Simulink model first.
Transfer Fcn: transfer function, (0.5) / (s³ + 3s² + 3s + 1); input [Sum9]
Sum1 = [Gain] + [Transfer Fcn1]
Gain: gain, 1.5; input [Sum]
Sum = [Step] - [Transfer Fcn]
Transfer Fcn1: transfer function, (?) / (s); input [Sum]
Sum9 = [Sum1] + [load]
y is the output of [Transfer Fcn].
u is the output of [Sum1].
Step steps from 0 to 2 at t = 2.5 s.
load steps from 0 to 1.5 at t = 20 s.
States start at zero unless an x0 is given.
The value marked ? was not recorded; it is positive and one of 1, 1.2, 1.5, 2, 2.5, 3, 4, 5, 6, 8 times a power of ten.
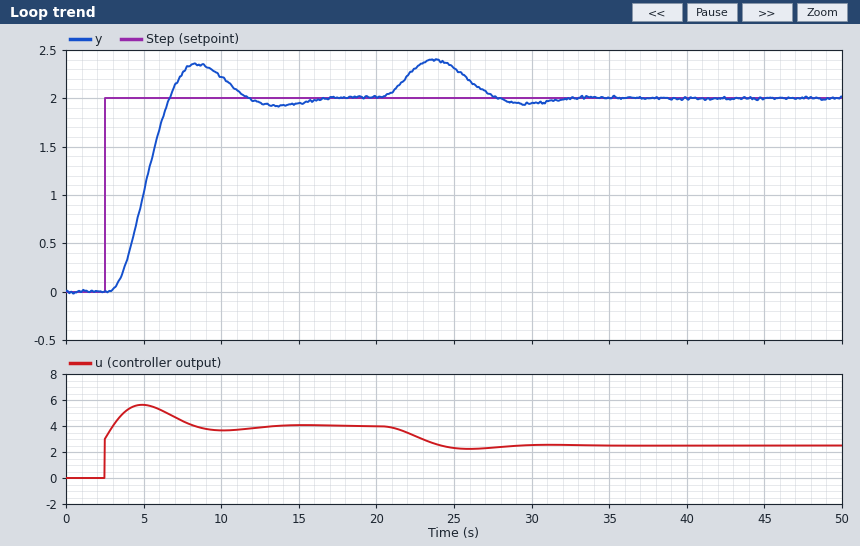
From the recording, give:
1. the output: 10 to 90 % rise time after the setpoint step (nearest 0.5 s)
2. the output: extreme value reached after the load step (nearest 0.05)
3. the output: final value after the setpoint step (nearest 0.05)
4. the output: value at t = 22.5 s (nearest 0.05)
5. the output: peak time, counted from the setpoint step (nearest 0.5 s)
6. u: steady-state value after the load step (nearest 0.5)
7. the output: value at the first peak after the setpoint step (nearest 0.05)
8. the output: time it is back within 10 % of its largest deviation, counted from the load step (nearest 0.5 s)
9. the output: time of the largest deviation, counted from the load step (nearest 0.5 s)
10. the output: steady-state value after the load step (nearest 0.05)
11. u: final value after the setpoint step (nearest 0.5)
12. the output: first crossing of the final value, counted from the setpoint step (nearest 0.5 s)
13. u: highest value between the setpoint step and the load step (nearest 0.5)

2.5 s
2.40
2.00
2.30
6.0 s
2.5
2.35
11.0 s
3.5 s
2.00
4.0
4.0 s
5.5
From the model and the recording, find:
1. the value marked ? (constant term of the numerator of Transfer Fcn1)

1
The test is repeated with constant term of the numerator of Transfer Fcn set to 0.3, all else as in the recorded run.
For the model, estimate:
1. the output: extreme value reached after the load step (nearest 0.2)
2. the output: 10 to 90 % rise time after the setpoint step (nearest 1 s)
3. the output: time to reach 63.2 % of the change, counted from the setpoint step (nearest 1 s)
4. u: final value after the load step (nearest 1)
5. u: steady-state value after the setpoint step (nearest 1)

2.2
4 s
4 s
5
7
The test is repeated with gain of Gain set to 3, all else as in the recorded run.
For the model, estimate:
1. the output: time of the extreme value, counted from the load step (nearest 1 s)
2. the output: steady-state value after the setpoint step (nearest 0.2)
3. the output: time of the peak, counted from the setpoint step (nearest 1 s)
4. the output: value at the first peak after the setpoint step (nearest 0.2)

3 s
2.0
4 s
2.2
